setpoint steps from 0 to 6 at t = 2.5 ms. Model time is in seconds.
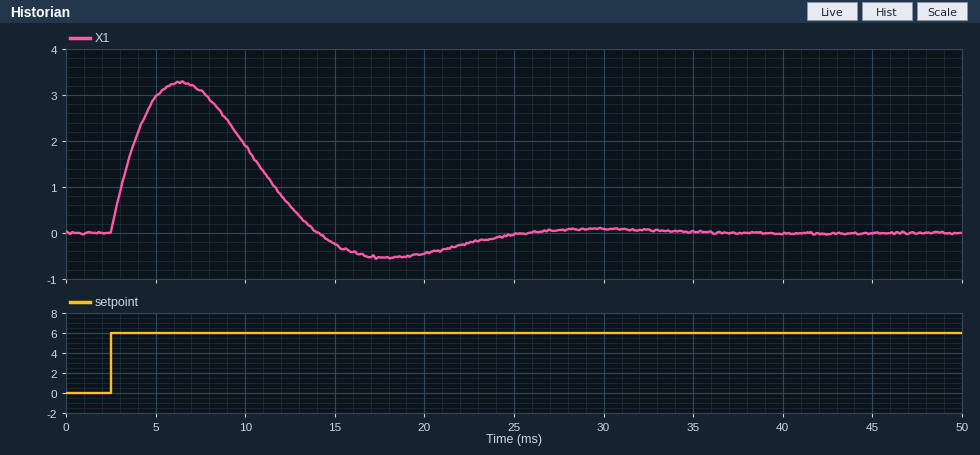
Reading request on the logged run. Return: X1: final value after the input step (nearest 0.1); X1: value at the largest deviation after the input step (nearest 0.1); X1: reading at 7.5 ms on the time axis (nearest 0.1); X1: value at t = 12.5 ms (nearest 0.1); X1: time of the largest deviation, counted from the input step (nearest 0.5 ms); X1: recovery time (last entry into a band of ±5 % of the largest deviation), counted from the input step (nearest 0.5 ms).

0.0
3.3
3.1
0.6
4.0 ms
20.5 ms
